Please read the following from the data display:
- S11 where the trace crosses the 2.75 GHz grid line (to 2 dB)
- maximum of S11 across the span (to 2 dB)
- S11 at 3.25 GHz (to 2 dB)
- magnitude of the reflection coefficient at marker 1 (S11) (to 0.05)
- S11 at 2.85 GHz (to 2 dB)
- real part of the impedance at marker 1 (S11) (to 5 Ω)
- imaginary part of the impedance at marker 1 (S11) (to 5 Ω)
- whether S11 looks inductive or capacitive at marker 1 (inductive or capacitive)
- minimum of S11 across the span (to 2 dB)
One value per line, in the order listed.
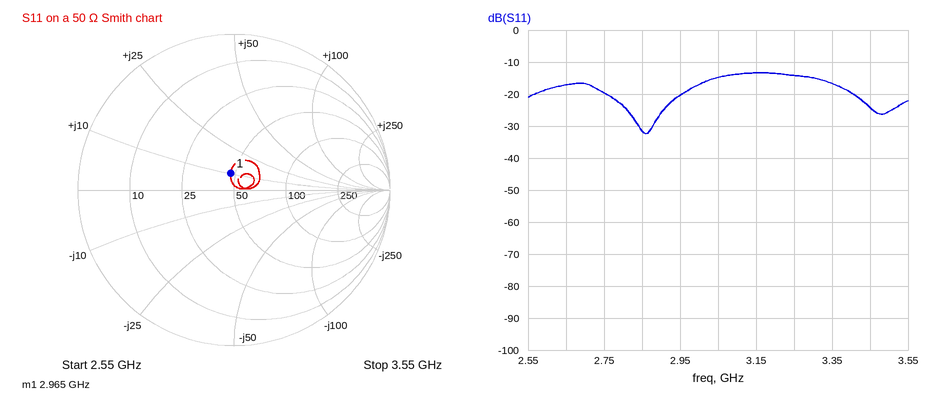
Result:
-20 dB
-14 dB
-14 dB
0.10
-32 dB
45 Ω
+10 Ω
inductive
-32 dB
